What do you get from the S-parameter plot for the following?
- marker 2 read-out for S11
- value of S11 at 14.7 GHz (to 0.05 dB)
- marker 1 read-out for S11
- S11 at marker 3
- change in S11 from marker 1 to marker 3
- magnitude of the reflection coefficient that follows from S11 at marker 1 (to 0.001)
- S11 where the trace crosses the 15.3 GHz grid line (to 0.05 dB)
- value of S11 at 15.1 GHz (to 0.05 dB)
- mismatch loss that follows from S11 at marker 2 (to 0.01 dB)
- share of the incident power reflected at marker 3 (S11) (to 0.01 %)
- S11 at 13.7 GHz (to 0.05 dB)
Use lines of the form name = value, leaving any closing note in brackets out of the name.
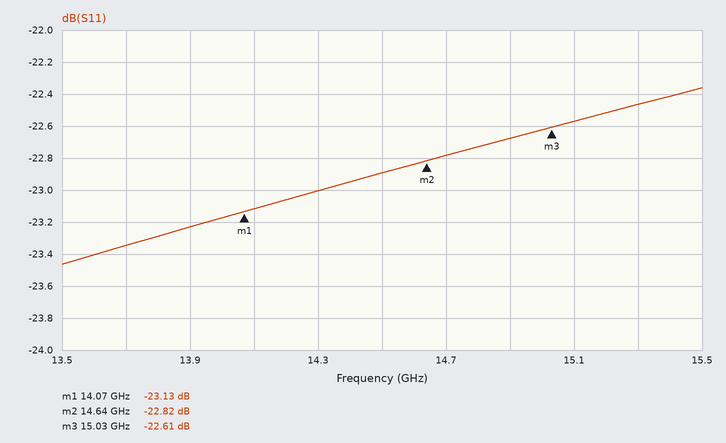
marker 2 read-out for S11 = -22.82 dB
value of S11 at 14.7 GHz = -22.80 dB
marker 1 read-out for S11 = -23.13 dB
S11 at marker 3 = -22.61 dB
change in S11 from marker 1 to marker 3 = 0.52 dB
magnitude of the reflection coefficient that follows from S11 at marker 1 = 0.070
S11 where the trace crosses the 15.3 GHz grid line = -22.45 dB
value of S11 at 15.1 GHz = -22.55 dB
mismatch loss that follows from S11 at marker 2 = 0.02 dB
share of the incident power reflected at marker 3 (S11) = 0.55 %
S11 at 13.7 GHz = -23.35 dB
